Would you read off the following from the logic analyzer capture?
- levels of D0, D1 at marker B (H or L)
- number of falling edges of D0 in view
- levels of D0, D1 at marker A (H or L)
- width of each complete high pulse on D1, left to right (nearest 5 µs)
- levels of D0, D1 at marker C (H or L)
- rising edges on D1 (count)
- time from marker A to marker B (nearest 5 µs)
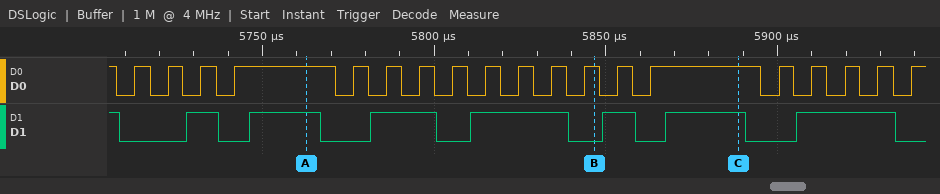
D0=H, D1=L
19
D0=H, D1=H
10 µs, 20 µs, 20 µs, 30 µs, 10 µs, 25 µs, 30 µs
D0=H, D1=H
7
85 µs
